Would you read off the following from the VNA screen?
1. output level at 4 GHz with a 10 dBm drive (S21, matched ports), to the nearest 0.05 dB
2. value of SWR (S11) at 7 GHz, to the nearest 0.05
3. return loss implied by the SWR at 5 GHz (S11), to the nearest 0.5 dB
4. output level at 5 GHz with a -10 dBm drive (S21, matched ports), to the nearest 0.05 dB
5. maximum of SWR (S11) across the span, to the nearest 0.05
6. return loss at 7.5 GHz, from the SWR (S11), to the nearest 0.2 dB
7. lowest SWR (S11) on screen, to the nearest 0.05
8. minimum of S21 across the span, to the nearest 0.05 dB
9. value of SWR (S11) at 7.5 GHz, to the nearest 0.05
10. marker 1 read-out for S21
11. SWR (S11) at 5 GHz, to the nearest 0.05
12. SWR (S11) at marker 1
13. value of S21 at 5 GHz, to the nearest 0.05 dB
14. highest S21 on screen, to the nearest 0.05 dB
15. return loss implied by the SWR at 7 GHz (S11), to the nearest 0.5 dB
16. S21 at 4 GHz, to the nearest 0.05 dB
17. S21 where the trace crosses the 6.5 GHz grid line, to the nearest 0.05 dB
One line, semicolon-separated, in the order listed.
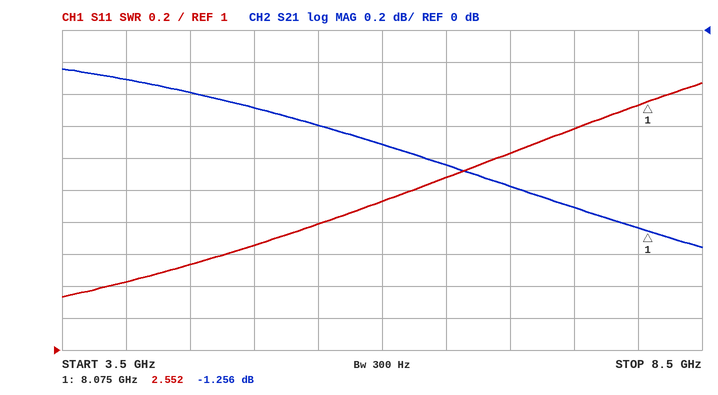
9.70 dBm; 2.25; 12.0 dB; -10.50 dBm; 2.65; 7.8 dB; 1.35; -1.35 dB; 2.40; -1.256 dB; 1.65; 2.552; -0.50 dB; -0.25 dB; 8.5 dB; -0.30 dB; -0.85 dB
